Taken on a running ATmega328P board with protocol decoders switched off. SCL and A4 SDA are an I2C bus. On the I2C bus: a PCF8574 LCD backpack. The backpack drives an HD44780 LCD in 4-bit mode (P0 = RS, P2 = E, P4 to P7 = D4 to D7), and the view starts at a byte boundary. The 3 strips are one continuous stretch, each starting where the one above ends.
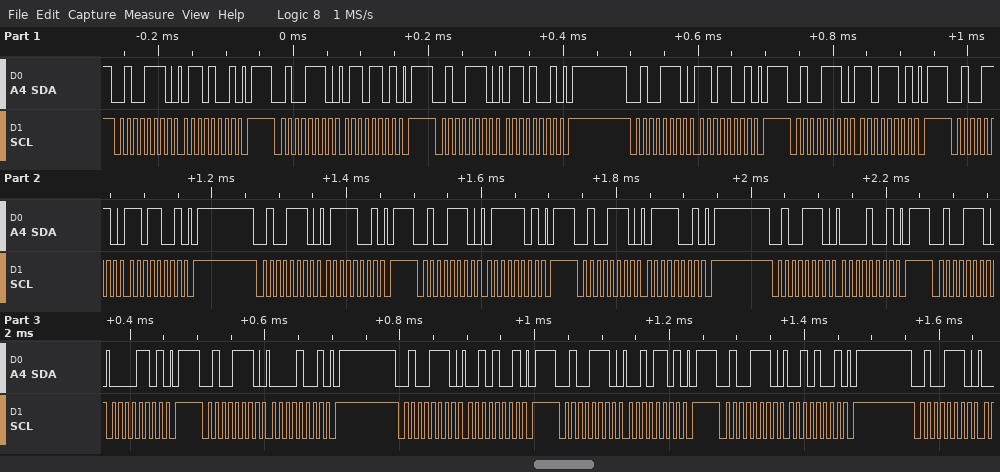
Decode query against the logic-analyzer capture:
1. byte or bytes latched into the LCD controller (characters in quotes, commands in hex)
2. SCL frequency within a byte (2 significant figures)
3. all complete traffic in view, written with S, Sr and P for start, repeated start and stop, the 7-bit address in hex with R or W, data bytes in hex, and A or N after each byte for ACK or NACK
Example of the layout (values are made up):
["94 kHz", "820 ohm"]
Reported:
["'m' 'p'", "100 kHz", "S 27W A 69 A P S 27W A 6D A P S 27W A 69 A P S 27W A D9 A P S 27W A DD A P S 27W A D9 A P S 27W A 79 A P S 27W A 7D A P S 27W A 79 A P S 27W A 09 A P S 27W A 0D A P S 27W A 09 A P S 27W A 29 A P S 27W A 2D A P S 27W A 29 A P S 27W A"]
